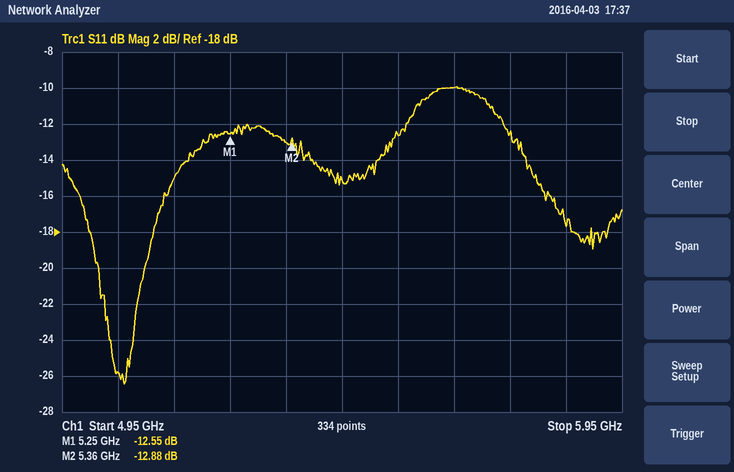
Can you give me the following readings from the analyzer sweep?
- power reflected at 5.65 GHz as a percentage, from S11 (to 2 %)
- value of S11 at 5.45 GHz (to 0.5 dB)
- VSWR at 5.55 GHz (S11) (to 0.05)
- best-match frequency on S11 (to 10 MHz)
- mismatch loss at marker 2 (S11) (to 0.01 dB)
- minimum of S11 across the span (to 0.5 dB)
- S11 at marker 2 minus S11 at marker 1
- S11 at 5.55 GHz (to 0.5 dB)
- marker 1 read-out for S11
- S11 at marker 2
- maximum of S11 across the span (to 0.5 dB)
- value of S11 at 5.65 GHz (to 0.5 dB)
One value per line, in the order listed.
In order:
10 %
-15.0 dB
1.60
5.06 GHz
0.23 dB
-26.5 dB
-0.33 dB
-12.5 dB
-12.55 dB
-12.88 dB
-10.0 dB
-10.0 dB
